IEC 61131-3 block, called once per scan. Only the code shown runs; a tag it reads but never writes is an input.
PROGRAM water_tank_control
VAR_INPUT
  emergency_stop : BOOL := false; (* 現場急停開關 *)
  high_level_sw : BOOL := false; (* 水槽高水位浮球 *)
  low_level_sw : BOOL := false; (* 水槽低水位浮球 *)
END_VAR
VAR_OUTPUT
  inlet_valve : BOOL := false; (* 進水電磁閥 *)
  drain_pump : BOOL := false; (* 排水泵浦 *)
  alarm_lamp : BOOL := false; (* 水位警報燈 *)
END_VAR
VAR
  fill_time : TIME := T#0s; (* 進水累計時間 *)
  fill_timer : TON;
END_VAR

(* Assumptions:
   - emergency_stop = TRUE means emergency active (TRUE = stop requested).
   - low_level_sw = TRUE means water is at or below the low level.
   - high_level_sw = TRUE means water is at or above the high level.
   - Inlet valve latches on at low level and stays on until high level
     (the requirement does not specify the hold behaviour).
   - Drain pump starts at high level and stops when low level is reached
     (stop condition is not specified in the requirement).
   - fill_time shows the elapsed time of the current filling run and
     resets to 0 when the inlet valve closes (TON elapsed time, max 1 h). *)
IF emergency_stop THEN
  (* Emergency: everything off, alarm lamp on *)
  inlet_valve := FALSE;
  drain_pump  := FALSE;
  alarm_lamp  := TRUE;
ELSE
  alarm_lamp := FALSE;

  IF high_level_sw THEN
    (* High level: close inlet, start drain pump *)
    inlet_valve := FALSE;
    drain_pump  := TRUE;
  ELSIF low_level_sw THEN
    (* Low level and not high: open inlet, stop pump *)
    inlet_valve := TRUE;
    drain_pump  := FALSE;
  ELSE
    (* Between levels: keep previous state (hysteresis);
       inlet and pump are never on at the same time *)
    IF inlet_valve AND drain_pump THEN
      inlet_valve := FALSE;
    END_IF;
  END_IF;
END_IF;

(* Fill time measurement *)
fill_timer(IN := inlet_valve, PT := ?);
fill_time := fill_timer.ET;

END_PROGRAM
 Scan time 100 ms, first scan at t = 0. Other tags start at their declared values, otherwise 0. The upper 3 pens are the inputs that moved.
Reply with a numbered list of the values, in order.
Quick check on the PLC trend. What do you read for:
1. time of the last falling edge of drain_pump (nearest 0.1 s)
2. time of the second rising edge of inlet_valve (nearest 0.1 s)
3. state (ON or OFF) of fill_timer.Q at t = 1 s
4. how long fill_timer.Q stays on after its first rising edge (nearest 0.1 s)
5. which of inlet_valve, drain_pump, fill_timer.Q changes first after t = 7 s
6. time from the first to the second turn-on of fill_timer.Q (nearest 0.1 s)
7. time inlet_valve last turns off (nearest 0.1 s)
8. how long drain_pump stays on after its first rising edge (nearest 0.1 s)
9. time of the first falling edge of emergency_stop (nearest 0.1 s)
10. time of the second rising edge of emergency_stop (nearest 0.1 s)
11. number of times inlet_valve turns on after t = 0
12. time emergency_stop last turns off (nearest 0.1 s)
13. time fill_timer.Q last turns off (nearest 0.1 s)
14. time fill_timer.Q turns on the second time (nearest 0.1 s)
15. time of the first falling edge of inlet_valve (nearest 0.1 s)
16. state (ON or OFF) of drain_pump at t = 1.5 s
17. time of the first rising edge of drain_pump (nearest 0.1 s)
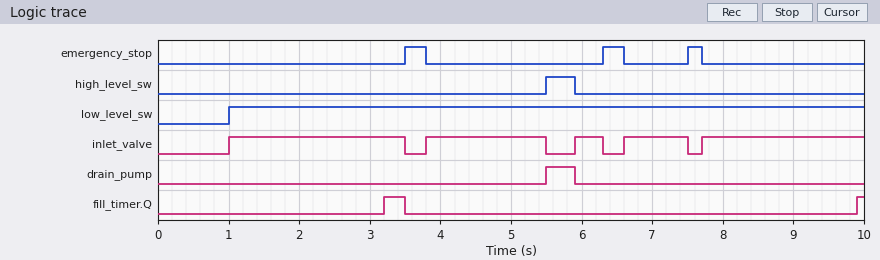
1. 5.9 s
2. 3.8 s
3. OFF
4. 0.3 s
5. inlet_valve
6. 6.7 s
7. 7.5 s
8. 0.4 s
9. 3.8 s
10. 6.3 s
11. 5
12. 7.7 s
13. 3.5 s
14. 9.9 s
15. 3.5 s
16. OFF
17. 5.5 s
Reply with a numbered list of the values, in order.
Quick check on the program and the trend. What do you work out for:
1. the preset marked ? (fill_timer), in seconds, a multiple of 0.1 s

1. 2.2 s
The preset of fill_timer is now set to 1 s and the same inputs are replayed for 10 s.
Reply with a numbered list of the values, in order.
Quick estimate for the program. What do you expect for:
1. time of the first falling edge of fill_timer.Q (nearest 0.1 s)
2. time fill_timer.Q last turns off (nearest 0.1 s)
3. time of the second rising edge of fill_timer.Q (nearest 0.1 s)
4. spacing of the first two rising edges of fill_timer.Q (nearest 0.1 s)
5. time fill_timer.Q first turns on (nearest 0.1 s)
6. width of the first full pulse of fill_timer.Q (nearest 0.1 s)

1. 3.5 s
2. 5.5 s
3. 4.8 s
4. 2.8 s
5. 2.0 s
6. 1.5 s
